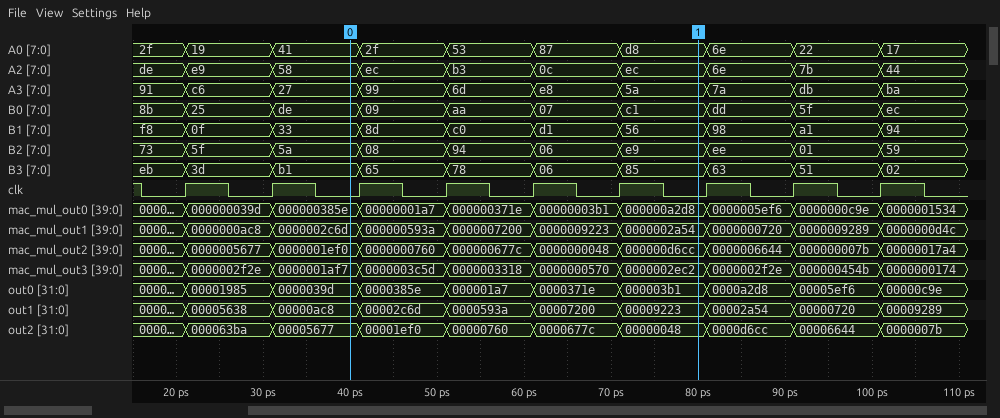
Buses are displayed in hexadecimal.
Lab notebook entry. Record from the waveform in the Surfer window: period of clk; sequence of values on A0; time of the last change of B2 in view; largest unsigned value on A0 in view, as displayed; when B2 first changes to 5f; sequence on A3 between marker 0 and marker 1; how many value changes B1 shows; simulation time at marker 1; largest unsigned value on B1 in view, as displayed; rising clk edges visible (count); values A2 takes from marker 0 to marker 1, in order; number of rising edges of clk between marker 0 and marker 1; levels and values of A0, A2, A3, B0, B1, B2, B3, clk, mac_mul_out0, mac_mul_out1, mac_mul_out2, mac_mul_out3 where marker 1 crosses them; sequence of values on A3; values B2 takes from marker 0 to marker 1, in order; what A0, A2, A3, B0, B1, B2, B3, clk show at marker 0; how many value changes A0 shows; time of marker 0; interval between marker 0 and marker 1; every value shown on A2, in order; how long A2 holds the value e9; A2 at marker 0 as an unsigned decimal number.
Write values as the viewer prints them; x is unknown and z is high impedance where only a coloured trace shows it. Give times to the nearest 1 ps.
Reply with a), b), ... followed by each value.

a) 10 ps
b) 2f, 19, 41, 2f, 53, 87, d8, 6e, 22, 17
c) 101 ps
d) d8
e) 21 ps
f) 27, 99, 6d, e8, 5a
g) 9
h) 80 ps
i) f8
j) 9
k) 58, ec, b3, 0c, ec
l) 4
m) A0=d8, A2=ec, A3=5a, B0=c1, B1=56, B2=e9, B3=85, clk=0, mac_mul_out0=000000a2d8, mac_mul_out1=0000002a54, mac_mul_out2=000000d6cc, mac_mul_out3=0000002ec2
n) 91, c6, 27, 99, 6d, e8, 5a, 7a, db, ba
o) 5a, 08, 94, 06, e9
p) A0=41, A2=58, A3=27, B0=de, B1=33, B2=5a, B3=b1, clk=0
q) 9
r) 40 ps
s) 40 ps
t) de, e9, 58, ec, b3, 0c, ec, 6e, 7b, 44
u) 10 ps
v) 88
